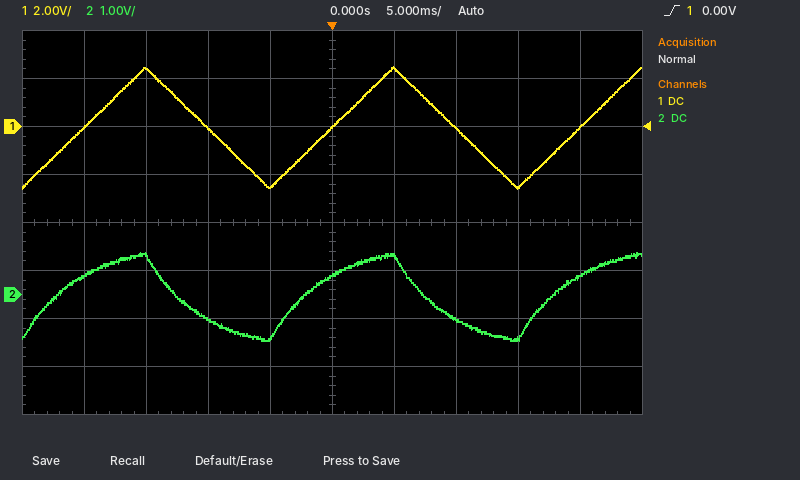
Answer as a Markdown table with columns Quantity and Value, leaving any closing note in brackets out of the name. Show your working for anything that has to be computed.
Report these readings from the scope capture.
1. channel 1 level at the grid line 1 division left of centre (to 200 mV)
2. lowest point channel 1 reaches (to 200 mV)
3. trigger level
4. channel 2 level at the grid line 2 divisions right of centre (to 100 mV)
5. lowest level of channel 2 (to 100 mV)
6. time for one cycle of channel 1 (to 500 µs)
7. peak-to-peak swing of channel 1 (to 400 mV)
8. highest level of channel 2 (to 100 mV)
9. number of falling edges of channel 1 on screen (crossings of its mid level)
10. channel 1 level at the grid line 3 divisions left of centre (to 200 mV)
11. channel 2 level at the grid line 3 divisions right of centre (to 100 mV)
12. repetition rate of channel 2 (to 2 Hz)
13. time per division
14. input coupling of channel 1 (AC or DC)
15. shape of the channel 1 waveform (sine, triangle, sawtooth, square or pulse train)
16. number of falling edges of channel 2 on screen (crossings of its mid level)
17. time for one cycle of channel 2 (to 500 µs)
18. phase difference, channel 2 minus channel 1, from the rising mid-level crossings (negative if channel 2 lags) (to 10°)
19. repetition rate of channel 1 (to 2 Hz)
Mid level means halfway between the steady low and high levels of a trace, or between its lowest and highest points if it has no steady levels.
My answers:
| Quantity | Value |
|---|---|
| channel 1 level at the grid line 1 division left of centre | -2.4 V |
| lowest point channel 1 reaches | -2.6 V |
| trigger level | 0.00 V |
| channel 2 level at the grid line 2 divisions right of centre | -500 mV |
| lowest level of channel 2 | -1.0 V |
| time for one cycle of channel 1 | 20.0 ms |
| peak-to-peak swing of channel 1 | 5.2 V |
| highest level of channel 2 | 900 mV |
| number of falling edges of channel 1 on screen | 2 |
| channel 1 level at the grid line 3 divisions left of centre | 2.4 V |
| channel 2 level at the grid line 3 divisions right of centre | -900 mV |
| repetition rate of channel 2 | 1 / 20.0 ms ≈ 50 Hz |
| time per division | 5 ms |
| input coupling of channel 1 | DC |
| shape of the channel 1 waveform | triangle |
| number of falling edges of channel 2 on screen | 2 |
| time for one cycle of channel 2 | 20.0 ms |
| phase difference, channel 2 minus channel 1, from the rising mid-level crossings (negative if channel 2 lags) | +40° |
| repetition rate of channel 1 | 1 / 20.0 ms ≈ 50 Hz |
